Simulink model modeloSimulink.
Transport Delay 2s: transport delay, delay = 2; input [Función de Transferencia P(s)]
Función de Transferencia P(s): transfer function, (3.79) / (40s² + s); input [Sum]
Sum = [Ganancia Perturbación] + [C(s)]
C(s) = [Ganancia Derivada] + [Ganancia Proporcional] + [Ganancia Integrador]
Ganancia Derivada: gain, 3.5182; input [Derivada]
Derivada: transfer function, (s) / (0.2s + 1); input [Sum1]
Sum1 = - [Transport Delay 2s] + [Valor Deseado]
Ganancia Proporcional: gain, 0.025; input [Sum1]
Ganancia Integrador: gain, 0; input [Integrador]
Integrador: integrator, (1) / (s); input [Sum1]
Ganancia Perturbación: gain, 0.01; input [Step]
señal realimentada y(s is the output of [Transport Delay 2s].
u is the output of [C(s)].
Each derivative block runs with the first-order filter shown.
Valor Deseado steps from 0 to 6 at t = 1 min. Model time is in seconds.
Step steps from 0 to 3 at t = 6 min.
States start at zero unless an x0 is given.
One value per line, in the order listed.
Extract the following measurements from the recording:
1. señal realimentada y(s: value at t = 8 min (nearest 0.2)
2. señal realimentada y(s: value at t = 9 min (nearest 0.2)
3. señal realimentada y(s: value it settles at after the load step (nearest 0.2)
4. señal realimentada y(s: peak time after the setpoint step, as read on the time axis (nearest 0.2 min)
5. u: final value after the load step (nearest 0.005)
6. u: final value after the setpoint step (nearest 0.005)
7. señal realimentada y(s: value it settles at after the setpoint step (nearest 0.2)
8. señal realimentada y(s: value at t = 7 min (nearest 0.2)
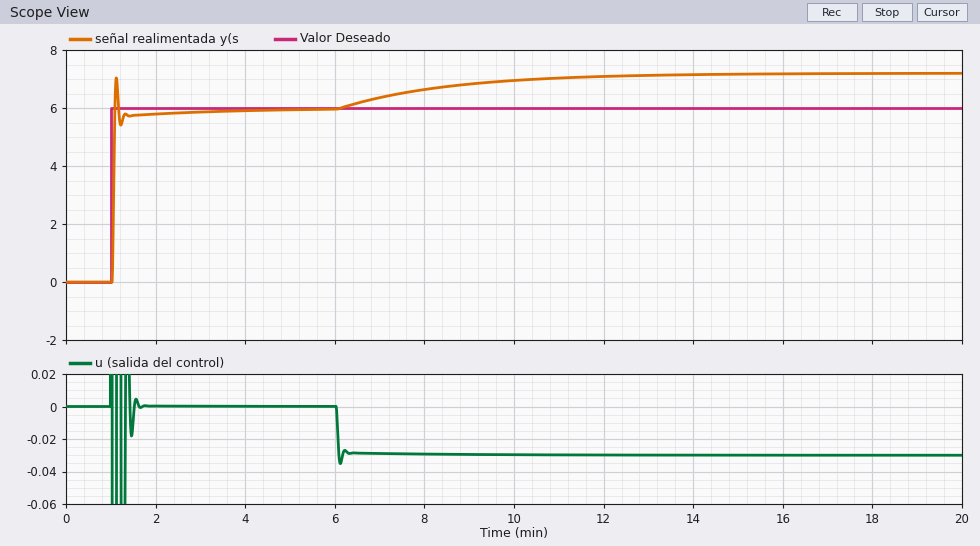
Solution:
6.6
6.8
7.2
1.2 min
-0.030
0.000
6.0
6.4
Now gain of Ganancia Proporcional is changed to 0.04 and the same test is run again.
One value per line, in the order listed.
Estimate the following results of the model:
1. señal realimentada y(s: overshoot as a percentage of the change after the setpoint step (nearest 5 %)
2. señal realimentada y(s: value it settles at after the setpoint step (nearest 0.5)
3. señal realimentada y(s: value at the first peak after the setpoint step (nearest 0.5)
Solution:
20 %
6.0
7.0
